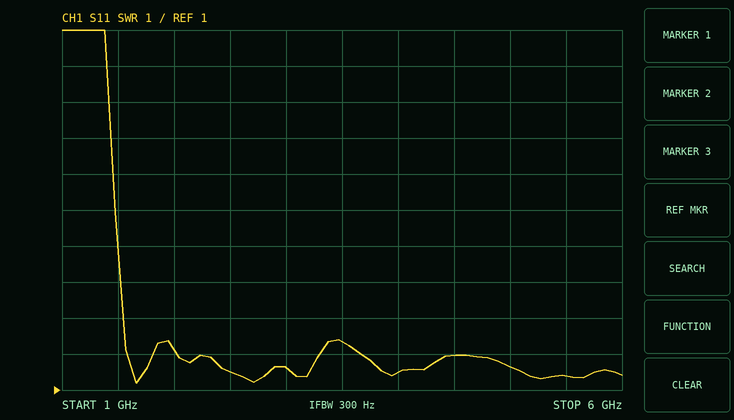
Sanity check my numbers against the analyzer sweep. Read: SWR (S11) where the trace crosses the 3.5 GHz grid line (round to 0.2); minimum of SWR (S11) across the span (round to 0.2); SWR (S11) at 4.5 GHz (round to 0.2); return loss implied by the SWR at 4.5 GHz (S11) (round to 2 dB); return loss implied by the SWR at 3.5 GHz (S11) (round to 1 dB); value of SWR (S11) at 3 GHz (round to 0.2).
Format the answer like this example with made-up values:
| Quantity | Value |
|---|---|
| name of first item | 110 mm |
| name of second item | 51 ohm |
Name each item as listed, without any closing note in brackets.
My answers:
| Quantity | Value |
|---|---|
| SWR (S11) where the trace crosses the 3.5 GHz grid line | 2.4 |
| minimum of SWR (S11) across the span | 1.2 |
| SWR (S11) at 4.5 GHz | 2.0 |
| return loss implied by the SWR at 4.5 GHz (S11) | 10 dB |
| return loss implied by the SWR at 3.5 GHz (S11) | 8 dB |
| value of SWR (S11) at 3 GHz | 1.6 |
